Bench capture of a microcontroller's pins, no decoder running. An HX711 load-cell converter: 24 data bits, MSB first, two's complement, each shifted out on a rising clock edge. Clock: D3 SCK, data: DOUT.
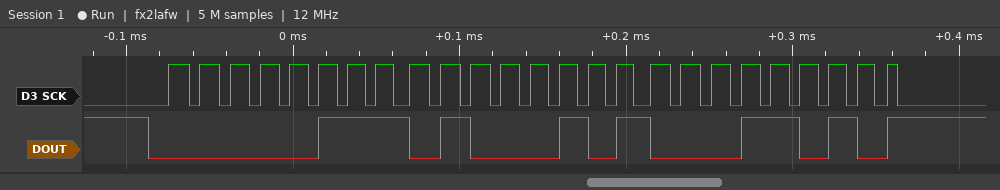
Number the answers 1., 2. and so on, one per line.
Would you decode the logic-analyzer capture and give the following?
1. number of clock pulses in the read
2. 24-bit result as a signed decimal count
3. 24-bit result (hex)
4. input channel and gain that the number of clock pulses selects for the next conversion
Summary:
1. 25
2. 476442
3. 0x07451A
4. channel A, gain 128
